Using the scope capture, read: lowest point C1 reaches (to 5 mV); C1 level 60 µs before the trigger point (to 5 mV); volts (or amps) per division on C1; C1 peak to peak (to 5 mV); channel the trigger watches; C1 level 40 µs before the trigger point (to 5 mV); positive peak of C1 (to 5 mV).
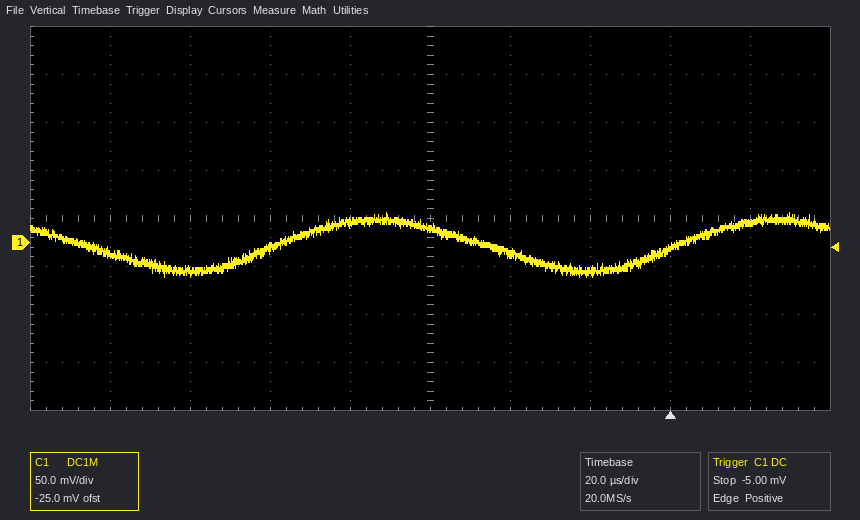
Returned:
-35 mV
15 mV
50 mV
65 mV
C1
-10 mV
30 mV
